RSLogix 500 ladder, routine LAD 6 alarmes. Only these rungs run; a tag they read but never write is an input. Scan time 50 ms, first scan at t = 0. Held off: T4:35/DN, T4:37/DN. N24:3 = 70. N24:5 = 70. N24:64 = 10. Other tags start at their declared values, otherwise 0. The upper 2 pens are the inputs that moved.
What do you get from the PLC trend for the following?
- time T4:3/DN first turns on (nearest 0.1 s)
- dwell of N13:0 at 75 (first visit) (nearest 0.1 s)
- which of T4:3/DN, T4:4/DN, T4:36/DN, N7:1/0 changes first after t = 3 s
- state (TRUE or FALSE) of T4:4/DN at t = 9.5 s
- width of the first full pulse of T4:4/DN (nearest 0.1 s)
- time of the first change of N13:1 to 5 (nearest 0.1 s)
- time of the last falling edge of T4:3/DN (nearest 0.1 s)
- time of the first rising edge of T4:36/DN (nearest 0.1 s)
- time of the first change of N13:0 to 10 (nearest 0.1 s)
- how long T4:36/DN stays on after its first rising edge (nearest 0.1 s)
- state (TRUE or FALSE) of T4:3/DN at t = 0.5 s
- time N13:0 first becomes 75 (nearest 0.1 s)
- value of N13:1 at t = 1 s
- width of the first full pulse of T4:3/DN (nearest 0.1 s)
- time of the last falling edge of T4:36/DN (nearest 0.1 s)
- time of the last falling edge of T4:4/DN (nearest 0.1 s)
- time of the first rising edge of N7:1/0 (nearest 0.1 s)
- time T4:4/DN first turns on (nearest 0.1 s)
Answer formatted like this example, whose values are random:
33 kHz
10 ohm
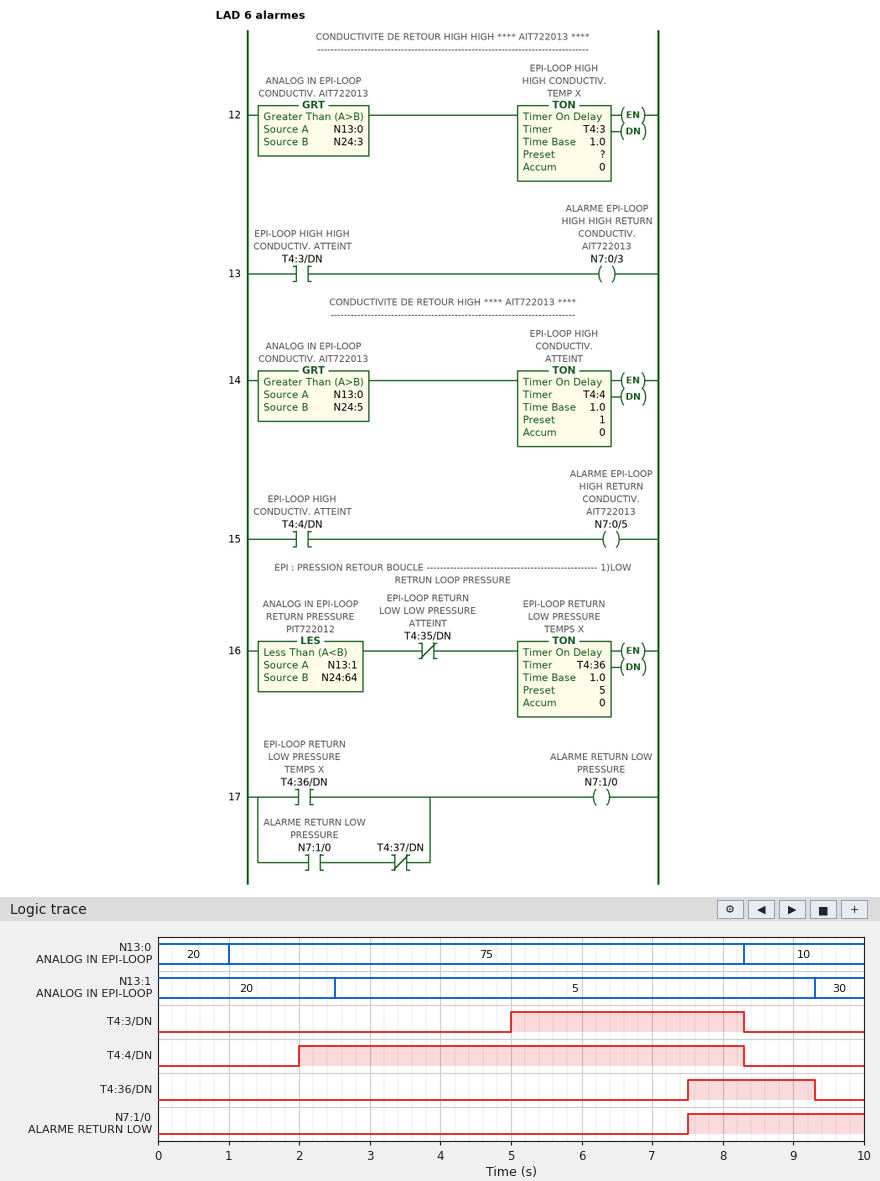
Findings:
5.0 s
7.3 s
T4:3/DN
FALSE
6.3 s
2.5 s
8.3 s
7.5 s
8.3 s
1.8 s
FALSE
1.0 s
20
3.3 s
9.3 s
8.3 s
7.5 s
2.0 s
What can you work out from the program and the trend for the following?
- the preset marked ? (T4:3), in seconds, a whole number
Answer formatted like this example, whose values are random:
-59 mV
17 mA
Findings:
4 s
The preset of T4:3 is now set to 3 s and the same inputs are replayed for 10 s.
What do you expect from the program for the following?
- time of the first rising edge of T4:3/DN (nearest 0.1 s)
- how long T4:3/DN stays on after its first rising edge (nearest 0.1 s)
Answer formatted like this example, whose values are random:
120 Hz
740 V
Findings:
4.0 s
4.3 s
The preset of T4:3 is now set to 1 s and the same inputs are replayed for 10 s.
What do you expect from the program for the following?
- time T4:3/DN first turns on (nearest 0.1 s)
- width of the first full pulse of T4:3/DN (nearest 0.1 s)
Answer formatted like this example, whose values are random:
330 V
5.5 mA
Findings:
2.0 s
6.3 s
